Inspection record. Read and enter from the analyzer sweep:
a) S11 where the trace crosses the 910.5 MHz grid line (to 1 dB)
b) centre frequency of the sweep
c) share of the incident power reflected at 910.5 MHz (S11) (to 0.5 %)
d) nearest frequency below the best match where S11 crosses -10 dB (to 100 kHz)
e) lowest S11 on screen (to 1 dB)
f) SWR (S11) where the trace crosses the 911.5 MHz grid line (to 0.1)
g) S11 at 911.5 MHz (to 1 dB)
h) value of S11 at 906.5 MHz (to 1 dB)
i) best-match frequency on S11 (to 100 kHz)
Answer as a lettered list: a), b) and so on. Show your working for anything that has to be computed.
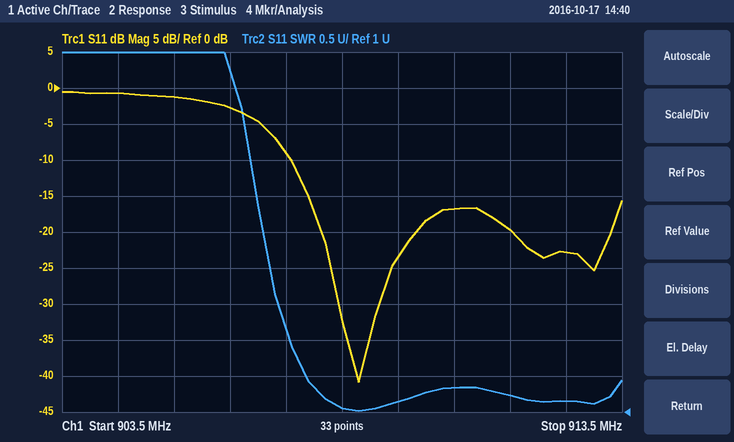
a) -17 dB
b) 908.5 MHz
c) 10^(-17/10) ≈ 2.0 %
d) 907.6 MHz
e) -41 dB
f) 1.2
g) -20 dB
h) -3 dB
i) 908.8 MHz
